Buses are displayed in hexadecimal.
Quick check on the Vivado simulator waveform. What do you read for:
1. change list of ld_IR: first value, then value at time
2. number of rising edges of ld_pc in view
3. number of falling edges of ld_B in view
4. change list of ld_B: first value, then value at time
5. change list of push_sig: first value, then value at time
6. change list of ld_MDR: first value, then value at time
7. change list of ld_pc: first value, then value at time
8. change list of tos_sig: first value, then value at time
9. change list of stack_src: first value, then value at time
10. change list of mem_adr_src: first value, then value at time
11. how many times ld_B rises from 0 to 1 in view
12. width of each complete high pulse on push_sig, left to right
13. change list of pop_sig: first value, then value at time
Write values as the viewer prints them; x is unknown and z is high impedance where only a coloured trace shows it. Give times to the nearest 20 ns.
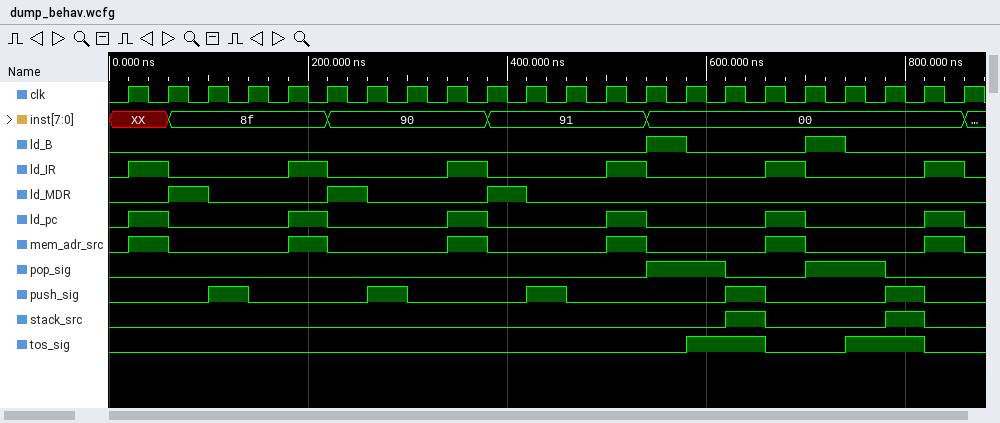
0, 1 at 20 ns, 0 at 60 ns, 1 at 180 ns, 0 at 220 ns, 1 at 340 ns, 0 at 380 ns, 1 at 500 ns, 0 at 540 ns, 1 at 660 ns, 0 at 700 ns, 1 at 820 ns, 0 at 860 ns
6
2
0, 1 at 540 ns, 0 at 580 ns, 1 at 700 ns, 0 at 740 ns
0, 1 at 100 ns, 0 at 140 ns, 1 at 260 ns, 0 at 300 ns, 1 at 420 ns, 0 at 460 ns, 1 at 620 ns, 0 at 660 ns, 1 at 780 ns, 0 at 820 ns
0, 1 at 60 ns, 0 at 100 ns, 1 at 220 ns, 0 at 260 ns, 1 at 380 ns, 0 at 420 ns
0, 1 at 20 ns, 0 at 60 ns, 1 at 180 ns, 0 at 220 ns, 1 at 340 ns, 0 at 380 ns, 1 at 500 ns, 0 at 540 ns, 1 at 660 ns, 0 at 700 ns, 1 at 820 ns, 0 at 860 ns
0, 1 at 580 ns, 0 at 660 ns, 1 at 740 ns, 0 at 820 ns
0, 1 at 620 ns, 0 at 660 ns, 1 at 780 ns, 0 at 820 ns
0, 1 at 20 ns, 0 at 60 ns, 1 at 180 ns, 0 at 220 ns, 1 at 340 ns, 0 at 380 ns, 1 at 500 ns, 0 at 540 ns, 1 at 660 ns, 0 at 700 ns, 1 at 820 ns, 0 at 860 ns
2
40 ns, 40 ns, 40 ns, 40 ns, 40 ns
0, 1 at 540 ns, 0 at 620 ns, 1 at 700 ns, 0 at 780 ns
